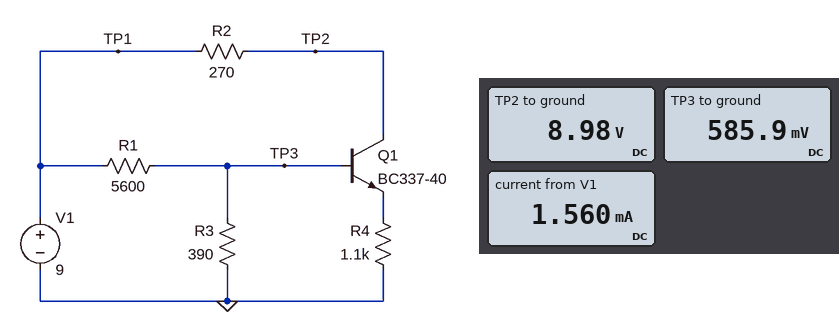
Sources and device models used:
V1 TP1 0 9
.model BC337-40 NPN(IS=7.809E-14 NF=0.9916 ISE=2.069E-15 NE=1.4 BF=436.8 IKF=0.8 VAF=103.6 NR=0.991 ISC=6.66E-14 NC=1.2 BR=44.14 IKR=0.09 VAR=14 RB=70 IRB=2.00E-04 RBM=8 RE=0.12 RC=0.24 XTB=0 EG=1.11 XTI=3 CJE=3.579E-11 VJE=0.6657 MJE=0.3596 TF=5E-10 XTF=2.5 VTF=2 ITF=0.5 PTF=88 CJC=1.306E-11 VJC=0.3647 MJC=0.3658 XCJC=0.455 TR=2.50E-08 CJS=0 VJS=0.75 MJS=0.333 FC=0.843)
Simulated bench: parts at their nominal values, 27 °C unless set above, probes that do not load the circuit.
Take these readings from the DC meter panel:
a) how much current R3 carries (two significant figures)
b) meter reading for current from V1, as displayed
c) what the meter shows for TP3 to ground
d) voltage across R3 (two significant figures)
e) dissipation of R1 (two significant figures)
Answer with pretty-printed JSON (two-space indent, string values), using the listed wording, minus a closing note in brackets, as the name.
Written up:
{
  "how much current R3 carries": "1.5 mA",
  "meter reading for current from V1, as displayed": "1.560 mA",
  "what the meter shows for TP3 to ground": "585.9 mV",
  "voltage across R3": "590 mV",
  "dissipation of R1": "13 mW"
}
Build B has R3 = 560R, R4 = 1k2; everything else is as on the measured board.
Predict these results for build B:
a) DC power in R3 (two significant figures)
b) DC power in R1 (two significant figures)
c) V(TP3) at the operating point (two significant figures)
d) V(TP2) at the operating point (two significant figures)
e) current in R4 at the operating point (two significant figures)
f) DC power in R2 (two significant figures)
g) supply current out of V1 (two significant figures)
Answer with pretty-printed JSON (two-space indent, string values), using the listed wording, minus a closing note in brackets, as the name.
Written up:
{
  "DC power in R3": "1.2 mW",
  "DC power in R1": "12 mW",
  "V(TP3) at the operating point": "820 mV",
  "V(TP2) at the operating point": "8.9 V",
  "current in R4 at the operating point": "220 µA",
  "DC power in R2": "13 µW",
  "supply current out of V1": "1.7 mA"
}
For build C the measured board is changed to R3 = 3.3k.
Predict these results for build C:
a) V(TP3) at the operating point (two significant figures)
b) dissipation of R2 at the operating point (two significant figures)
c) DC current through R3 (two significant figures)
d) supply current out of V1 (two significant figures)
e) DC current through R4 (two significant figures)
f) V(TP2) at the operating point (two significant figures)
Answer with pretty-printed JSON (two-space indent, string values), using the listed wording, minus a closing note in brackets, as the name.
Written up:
{
  "V(TP3) at the operating point": "3.3 V",
  "dissipation of R2 at the operating point": "1.6 mW",
  "DC current through R3": "1.0 mA",
  "supply current out of V1": "3.5 mA",
  "DC current through R4": "2.5 mA",
  "V(TP2) at the operating point": "8.3 V"
}
